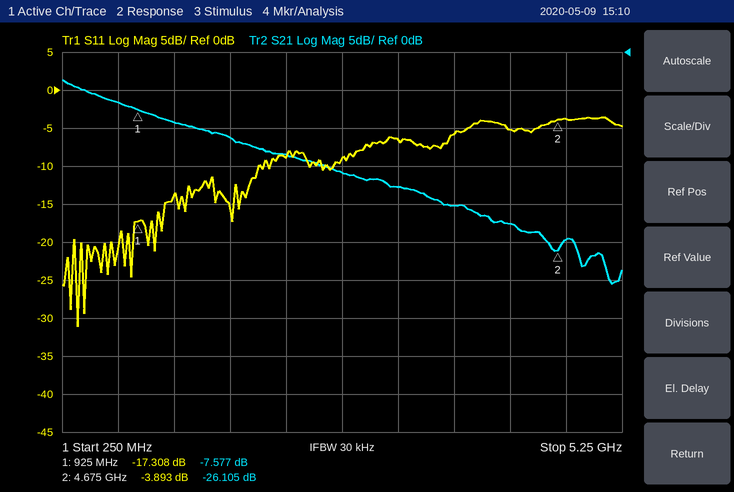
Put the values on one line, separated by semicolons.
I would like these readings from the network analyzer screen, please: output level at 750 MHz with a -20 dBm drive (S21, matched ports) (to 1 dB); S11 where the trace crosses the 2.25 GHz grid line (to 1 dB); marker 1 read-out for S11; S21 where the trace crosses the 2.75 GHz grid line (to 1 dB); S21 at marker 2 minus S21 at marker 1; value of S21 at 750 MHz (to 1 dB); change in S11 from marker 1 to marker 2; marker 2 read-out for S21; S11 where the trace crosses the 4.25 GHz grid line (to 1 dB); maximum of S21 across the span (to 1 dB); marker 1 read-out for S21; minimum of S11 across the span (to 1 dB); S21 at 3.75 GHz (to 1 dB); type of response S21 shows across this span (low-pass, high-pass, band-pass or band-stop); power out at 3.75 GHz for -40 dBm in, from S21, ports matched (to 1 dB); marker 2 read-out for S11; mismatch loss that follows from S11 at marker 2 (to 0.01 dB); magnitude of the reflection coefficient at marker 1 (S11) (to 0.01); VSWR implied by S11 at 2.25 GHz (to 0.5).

-27 dBm; -9 dB; -17.308 dB; -16 dB; -18.528 dB; -7 dB; 13.415 dB; -26.105 dB; -5 dB; -4 dB; -7.577 dB; -31 dB; -20 dB; low-pass; -60 dBm; -3.893 dB; 2.28 dB; 0.14; 2.0
